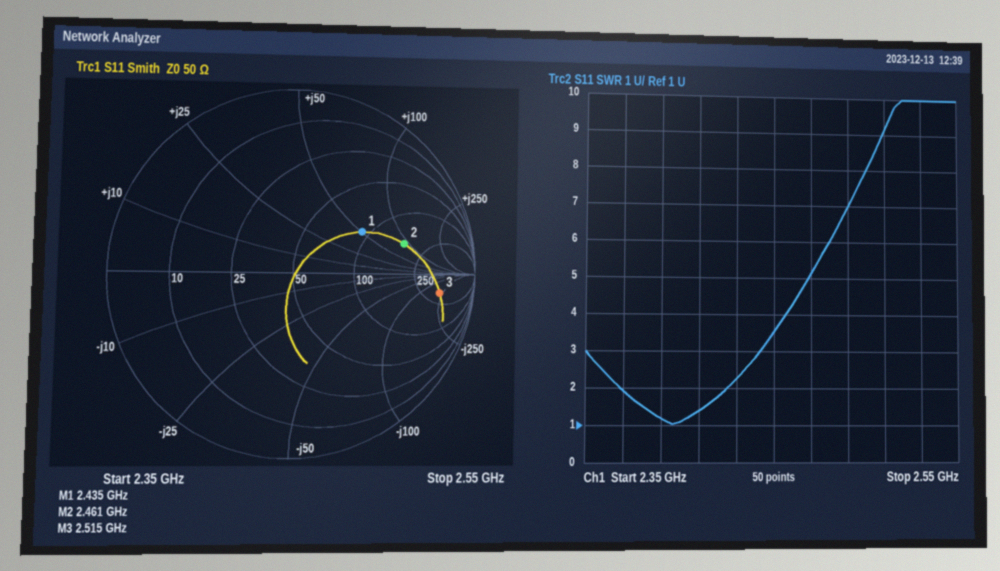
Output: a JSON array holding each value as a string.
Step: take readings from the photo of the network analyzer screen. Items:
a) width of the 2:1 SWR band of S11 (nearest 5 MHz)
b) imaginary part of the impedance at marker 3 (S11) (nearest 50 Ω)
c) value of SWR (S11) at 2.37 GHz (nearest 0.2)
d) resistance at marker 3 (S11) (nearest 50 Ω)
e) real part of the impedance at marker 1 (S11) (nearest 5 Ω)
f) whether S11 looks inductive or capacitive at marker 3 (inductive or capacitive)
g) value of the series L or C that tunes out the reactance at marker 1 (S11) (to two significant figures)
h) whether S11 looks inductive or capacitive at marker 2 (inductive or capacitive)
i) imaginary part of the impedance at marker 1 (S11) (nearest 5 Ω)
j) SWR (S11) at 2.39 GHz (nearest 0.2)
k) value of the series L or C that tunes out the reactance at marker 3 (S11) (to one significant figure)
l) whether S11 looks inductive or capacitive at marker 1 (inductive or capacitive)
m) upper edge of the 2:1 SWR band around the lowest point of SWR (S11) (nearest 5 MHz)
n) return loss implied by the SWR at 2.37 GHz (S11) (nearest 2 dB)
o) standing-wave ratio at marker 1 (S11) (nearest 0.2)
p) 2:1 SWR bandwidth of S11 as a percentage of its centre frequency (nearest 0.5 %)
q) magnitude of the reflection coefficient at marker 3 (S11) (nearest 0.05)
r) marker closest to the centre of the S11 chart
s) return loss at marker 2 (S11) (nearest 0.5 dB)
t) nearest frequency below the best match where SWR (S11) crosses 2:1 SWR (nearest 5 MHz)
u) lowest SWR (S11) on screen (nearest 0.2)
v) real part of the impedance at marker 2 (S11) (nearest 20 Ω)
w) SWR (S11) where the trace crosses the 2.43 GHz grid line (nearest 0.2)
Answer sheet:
["55 MHz", "-200 Ω", "2.0", "350 Ω", "90 Ω", "capacitive", "1.3 pF", "inductive", "+50 Ω", "1.2", "10 nH", "inductive", "2.425 GHz", "10 dB", "2.6", "2.5 %", "0.80", "marker 1", "4.0 dB", "2.370 GHz", "1.0", "160 Ω", "2.2"]
